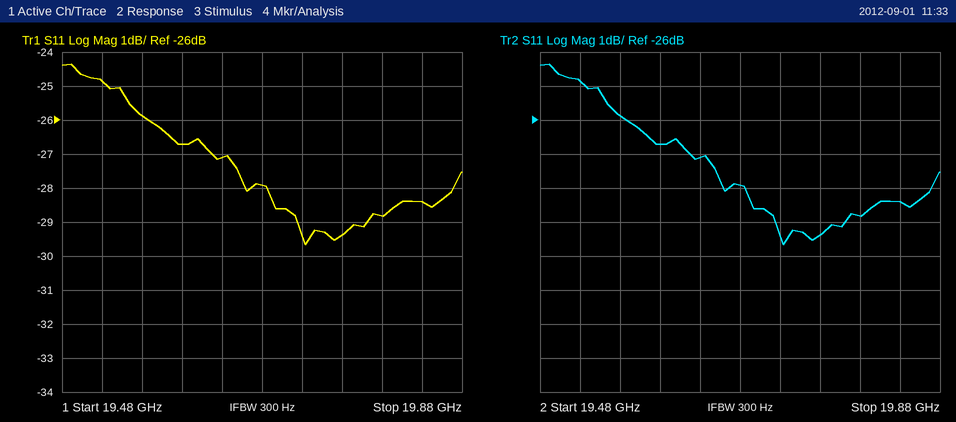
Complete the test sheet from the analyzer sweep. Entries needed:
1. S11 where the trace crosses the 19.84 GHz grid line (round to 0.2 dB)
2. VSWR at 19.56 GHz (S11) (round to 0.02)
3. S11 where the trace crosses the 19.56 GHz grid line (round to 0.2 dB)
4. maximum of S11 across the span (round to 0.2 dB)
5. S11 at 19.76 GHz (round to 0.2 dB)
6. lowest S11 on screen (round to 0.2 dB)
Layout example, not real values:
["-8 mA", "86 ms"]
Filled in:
["-28.4 dB", "1.10", "-25.8 dB", "-24.4 dB", "-29.4 dB", "-29.6 dB"]
